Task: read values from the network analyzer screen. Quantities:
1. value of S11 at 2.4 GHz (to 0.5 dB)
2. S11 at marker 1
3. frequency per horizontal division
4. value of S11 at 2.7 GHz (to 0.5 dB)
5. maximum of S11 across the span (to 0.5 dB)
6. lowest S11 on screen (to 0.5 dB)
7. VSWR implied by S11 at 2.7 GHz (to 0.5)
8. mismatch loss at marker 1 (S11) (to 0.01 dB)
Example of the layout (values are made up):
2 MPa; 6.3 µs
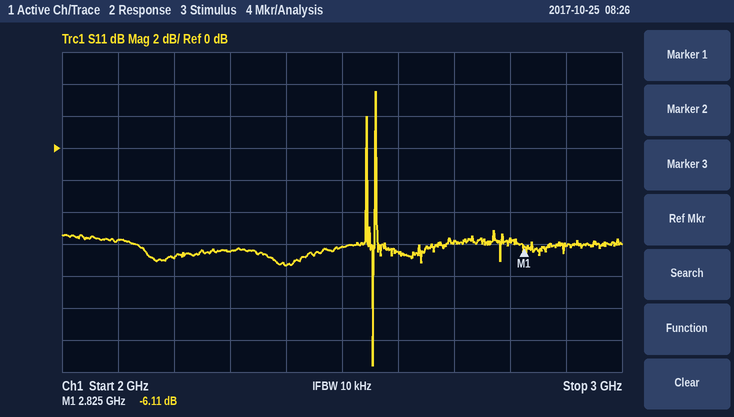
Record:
-7.5 dB; -6.11 dB; 100 MHz; -6.0 dB; 3.5 dB; -13.5 dB; 3.0; 1.22 dB
